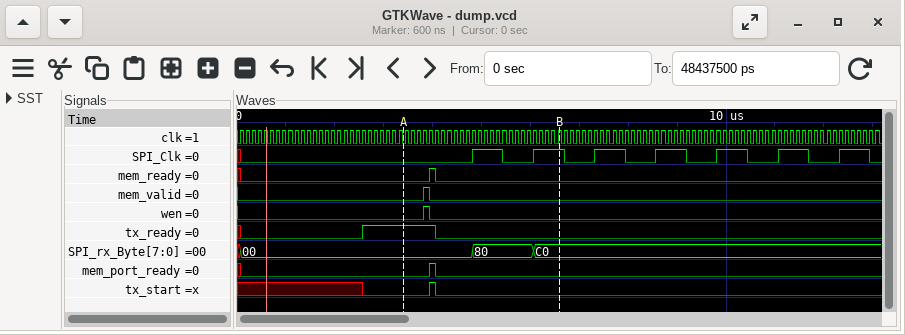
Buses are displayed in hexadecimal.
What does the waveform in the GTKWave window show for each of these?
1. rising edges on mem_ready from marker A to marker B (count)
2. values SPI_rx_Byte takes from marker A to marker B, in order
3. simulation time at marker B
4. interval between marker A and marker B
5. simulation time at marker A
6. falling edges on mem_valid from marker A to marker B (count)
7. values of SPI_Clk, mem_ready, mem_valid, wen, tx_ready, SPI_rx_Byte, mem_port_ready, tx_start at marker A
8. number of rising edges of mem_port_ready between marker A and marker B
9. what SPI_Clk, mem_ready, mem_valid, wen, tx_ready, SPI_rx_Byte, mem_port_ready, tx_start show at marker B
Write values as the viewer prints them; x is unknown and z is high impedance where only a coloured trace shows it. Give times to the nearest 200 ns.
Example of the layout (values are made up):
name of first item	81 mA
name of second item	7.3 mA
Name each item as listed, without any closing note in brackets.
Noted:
rising edges on mem_ready from marker A to marker B	1
values SPI_rx_Byte takes from marker A to marker B, in order	00, 80, C0
simulation time at marker B	6600 ns
interval between marker A and marker B	3200 ns
simulation time at marker A	3400 ns
falling edges on mem_valid from marker A to marker B	1
values of SPI_Clk, mem_ready, mem_valid, wen, tx_ready, SPI_rx_Byte, mem_port_ready, tx_start at marker A	SPI_Clk=0, mem_ready=0, mem_valid=0, wen=0, tx_ready=1, SPI_rx_Byte=00, mem_port_ready=0, tx_start=0
number of rising edges of mem_port_ready between marker A and marker B	1
what SPI_Clk, mem_ready, mem_valid, wen, tx_ready, SPI_rx_Byte, mem_port_ready, tx_start show at marker B	SPI_Clk=1, mem_ready=0, mem_valid=0, wen=0, tx_ready=0, SPI_rx_Byte=C0, mem_port_ready=0, tx_start=0
